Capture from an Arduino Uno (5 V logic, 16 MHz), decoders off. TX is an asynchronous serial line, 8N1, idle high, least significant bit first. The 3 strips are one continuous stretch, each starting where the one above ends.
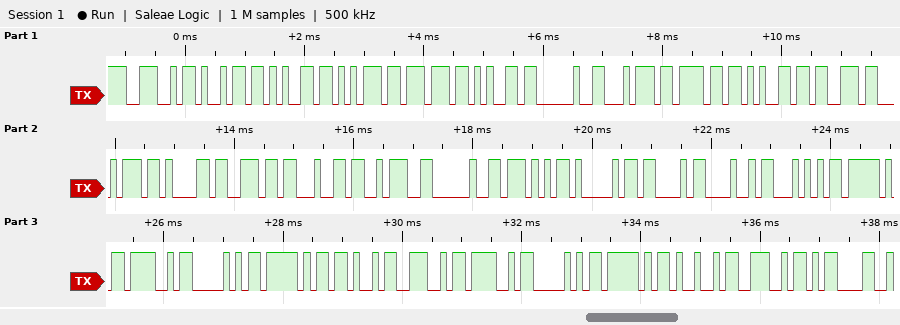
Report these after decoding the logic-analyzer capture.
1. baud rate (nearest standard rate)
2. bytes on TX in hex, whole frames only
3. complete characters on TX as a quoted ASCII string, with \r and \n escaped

9600 baud
4E 69 65 75 77 65 20 74 6F 65 73 74 61 6E 64 3A 20 57 41 43 48 54 5F 4F 50 5F 4B 4E 4F 50 5F 49 4E 0D
"Nieuwe toestand: WACHT_OP_KNOP_IN\r"
